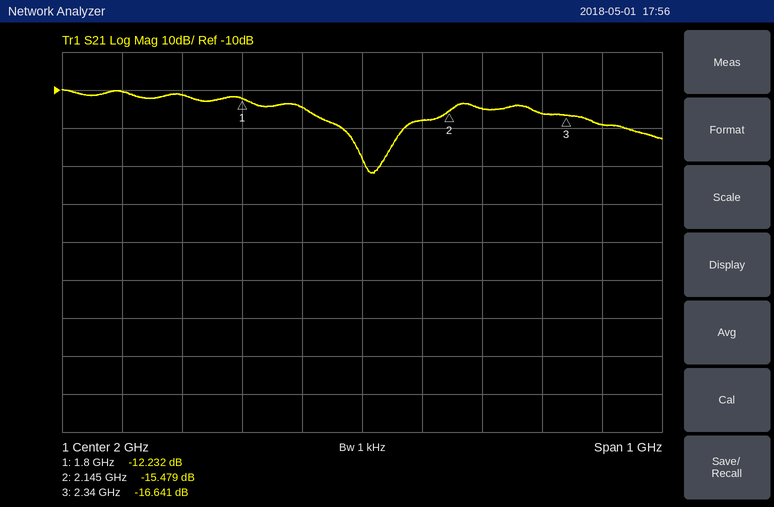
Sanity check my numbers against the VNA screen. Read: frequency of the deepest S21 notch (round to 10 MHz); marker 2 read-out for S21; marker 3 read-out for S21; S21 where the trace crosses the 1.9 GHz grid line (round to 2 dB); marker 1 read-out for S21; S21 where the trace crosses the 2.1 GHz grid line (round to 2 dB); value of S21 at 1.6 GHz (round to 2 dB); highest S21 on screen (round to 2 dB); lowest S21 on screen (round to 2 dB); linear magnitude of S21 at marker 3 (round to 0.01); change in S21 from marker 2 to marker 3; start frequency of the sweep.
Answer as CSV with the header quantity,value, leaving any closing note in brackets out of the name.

quantity,value
frequency of the deepest S21 notch,2.02 GHz
marker 2 read-out for S21,-15.479 dB
marker 3 read-out for S21,-16.641 dB
S21 where the trace crosses the 1.9 GHz grid line,-14 dB
marker 1 read-out for S21,-12.232 dB
S21 where the trace crosses the 2.1 GHz grid line,-18 dB
value of S21 at 1.6 GHz,-10 dB
highest S21 on screen,-10 dB
lowest S21 on screen,-32 dB
linear magnitude of S21 at marker 3,0.15
change in S21 from marker 2 to marker 3,-1.162 dB
start frequency of the sweep,1.5 GHz
